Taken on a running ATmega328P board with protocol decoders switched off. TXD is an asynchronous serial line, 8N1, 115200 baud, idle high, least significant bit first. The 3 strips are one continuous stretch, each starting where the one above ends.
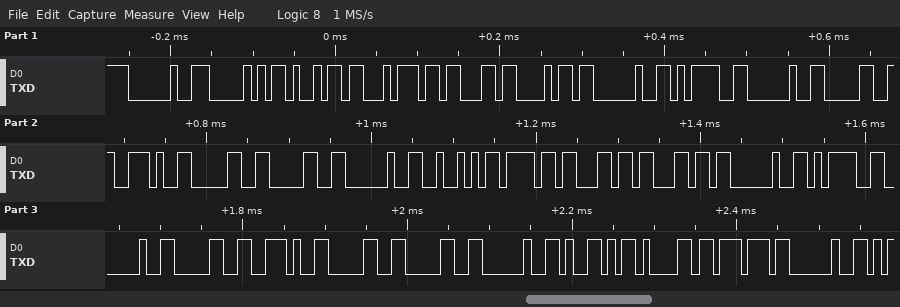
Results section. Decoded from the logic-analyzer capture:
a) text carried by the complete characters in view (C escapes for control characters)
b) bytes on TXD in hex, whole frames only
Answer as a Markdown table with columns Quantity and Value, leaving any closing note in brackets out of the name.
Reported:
| Quantity | Value |
|---|---|
| text carried by the complete characters in view | " Pitch = 0.00 Roll = 0.00 Yaw " |
| bytes on TXD in hex, whole frames only | 20 50 69 74 63 68 20 3D 20 30 2E 30 30 20 52 6F 6C 6C 20 3D 20 30 2E 30 30 20 59 61 77 20 |
